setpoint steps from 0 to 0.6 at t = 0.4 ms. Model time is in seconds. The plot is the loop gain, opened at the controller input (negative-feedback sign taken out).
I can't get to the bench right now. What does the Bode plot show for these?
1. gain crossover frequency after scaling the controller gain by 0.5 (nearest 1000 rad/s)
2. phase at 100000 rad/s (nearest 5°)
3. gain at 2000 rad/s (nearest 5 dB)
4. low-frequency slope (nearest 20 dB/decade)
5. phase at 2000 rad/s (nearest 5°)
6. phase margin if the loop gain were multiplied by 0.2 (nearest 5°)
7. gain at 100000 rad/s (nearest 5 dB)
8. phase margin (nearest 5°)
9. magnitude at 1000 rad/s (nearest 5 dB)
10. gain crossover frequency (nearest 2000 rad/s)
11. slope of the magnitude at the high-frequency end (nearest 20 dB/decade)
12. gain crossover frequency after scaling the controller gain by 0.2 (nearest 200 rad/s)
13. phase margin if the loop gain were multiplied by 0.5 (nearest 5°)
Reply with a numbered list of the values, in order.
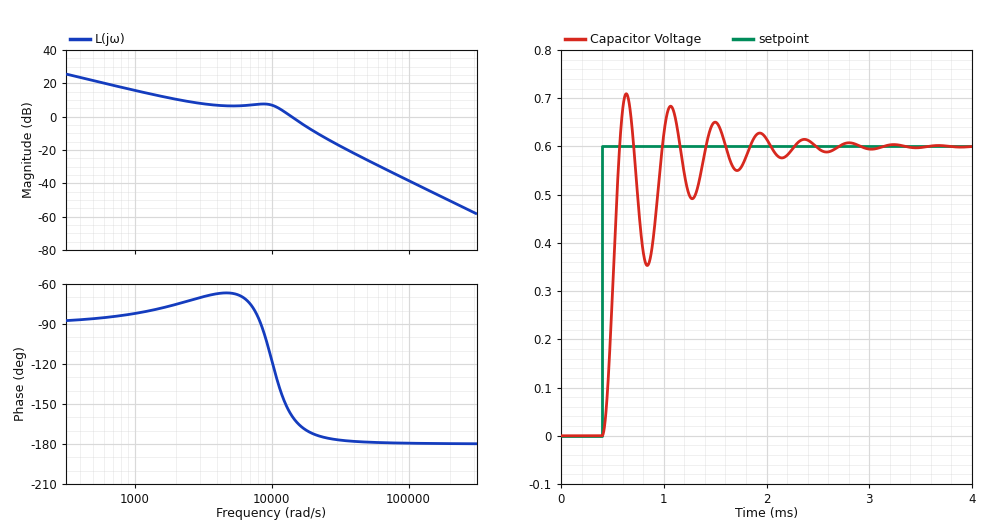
1. 11000 rad/s
2. -180°
3. 10 dB
4. -20 dB/decade
5. -75°
6. 100°
7. -40 dB
8. 20°
9. 15 dB
10. 14000 rad/s
11. -40 dB/decade
12. 1200 rad/s
13. 50°
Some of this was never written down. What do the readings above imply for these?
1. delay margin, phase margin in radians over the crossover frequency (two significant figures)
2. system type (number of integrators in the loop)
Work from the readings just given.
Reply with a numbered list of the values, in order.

1. 0.000025 s
2. 1
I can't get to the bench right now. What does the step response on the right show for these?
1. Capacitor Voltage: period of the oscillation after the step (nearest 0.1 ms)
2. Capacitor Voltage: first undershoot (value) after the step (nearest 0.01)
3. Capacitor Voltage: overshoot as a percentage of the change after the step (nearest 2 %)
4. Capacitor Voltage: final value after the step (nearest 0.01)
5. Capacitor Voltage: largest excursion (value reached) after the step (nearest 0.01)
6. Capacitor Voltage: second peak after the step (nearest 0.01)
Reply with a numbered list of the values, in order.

1. 0.4 ms
2. 0.35
3. 18 %
4. 0.60
5. 0.71
6. 0.68
